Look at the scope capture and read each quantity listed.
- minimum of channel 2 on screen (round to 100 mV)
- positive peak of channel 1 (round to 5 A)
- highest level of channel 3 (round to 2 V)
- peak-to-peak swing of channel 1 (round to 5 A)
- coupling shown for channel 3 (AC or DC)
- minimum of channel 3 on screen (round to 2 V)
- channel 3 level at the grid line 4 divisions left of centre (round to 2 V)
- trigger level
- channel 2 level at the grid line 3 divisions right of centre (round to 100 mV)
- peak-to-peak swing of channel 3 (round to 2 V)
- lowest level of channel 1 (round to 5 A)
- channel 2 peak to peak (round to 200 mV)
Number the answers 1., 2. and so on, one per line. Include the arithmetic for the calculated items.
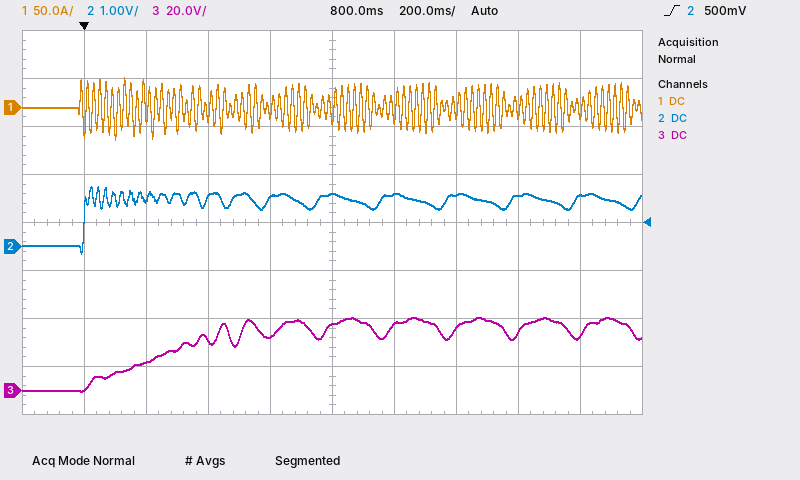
1. -100 mV
2. 30 A
3. 30 V
4. 30 A − (-35 A) = 65 A
5. DC
6. 0 V
7. 0 V
8. 500 mV
9. 1.1 V
10. 30 V − (0 V) = 30 V
11. -35 A
12. 1.4 V
